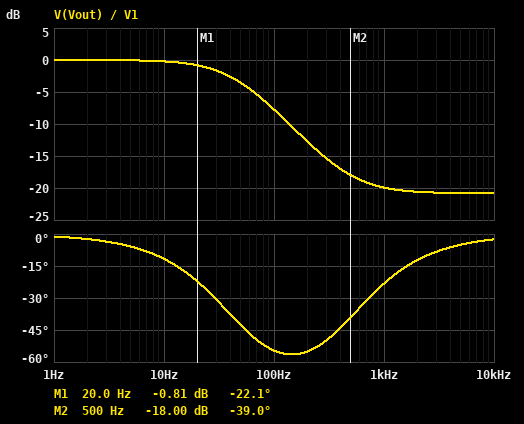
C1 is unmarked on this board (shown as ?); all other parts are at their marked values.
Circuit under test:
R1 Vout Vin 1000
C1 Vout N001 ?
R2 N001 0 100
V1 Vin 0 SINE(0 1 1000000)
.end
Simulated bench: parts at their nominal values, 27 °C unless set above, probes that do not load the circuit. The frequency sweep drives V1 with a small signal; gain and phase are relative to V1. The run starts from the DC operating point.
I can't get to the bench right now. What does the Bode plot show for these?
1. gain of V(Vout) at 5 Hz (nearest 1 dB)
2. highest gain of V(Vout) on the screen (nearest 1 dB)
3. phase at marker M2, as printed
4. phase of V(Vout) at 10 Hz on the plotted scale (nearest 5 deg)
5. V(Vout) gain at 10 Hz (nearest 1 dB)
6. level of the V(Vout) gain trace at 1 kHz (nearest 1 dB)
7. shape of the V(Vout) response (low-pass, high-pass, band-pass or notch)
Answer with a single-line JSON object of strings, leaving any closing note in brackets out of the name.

{"gain of V(Vout) at 5 Hz": "0 dB", "highest gain of V(Vout) on the screen": "0 dB", "phase at marker M2, as printed": "-39.0 deg", "phase of V(Vout) at 10 Hz on the plotted scale": "-10 deg", "V(Vout) gain at 10 Hz": "0 dB", "level of the V(Vout) gain trace at 1 kHz": "-20 dB", "shape of the V(Vout) response": "low-pass"}
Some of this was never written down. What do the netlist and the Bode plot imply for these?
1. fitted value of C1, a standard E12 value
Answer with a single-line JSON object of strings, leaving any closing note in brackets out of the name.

{"fitted value of C1, a standard E12 value": "3.3 µF"}
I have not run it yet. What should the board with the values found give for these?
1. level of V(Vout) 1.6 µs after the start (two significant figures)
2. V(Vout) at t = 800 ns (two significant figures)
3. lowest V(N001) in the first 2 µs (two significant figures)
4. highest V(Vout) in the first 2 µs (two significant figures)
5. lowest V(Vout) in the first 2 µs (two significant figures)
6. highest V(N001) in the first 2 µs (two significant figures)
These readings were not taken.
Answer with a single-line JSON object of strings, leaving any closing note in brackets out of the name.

{"level of V(Vout) 1.6 µs after the start": "-53 mV", "V(Vout) at t = 800 ns": "-86 mV", "lowest V(N001) in the first 2 µs": "-91 mV", "highest V(Vout) in the first 2 µs": "91 mV", "lowest V(Vout) in the first 2 µs": "-91 mV", "highest V(N001) in the first 2 µs": "91 mV"}
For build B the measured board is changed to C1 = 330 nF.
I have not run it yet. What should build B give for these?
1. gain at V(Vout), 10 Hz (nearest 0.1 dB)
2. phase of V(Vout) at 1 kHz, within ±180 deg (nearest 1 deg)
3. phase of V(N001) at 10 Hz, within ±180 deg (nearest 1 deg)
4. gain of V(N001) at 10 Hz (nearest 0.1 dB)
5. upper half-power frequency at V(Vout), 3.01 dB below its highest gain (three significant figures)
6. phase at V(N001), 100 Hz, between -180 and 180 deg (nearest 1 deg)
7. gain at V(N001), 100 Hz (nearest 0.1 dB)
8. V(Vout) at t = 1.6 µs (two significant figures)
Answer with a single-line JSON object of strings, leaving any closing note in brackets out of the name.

{"gain at V(Vout), 10 Hz": "0 dB", "phase of V(Vout) at 1 kHz, within ±180 deg": "-55 deg", "phase of V(N001) at 10 Hz, within ±180 deg": "89 deg", "gain of V(N001) at 10 Hz": "-53.7 dB", "upper half-power frequency at V(Vout), 3.01 dB below its highest gain": "442 Hz", "phase at V(N001), 100 Hz, between -180 and 180 deg": "77 deg", "gain at V(N001), 100 Hz": "-33.9 dB", "V(Vout) at t = 1.6 µs": "-53 mV"}
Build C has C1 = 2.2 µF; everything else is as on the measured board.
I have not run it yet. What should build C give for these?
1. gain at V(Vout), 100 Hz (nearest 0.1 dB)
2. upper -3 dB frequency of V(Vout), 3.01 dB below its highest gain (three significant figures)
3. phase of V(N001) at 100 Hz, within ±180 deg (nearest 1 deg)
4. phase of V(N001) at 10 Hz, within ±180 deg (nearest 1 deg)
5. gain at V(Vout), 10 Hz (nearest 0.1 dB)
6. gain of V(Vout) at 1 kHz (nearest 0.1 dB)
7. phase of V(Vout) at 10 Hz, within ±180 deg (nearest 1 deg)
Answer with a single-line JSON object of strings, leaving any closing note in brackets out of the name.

{"gain at V(Vout), 100 Hz": "-5.1 dB", "upper -3 dB frequency of V(Vout), 3.01 dB below its highest gain": "66.3 Hz", "phase of V(N001) at 100 Hz, within ±180 deg": "33 deg", "phase of V(N001) at 10 Hz, within ±180 deg": "81 deg", "gain at V(Vout), 10 Hz": "-0.1 dB", "gain of V(Vout) at 1 kHz": "-19.0 dB", "phase of V(Vout) at 10 Hz, within ±180 deg": "-8 deg"}
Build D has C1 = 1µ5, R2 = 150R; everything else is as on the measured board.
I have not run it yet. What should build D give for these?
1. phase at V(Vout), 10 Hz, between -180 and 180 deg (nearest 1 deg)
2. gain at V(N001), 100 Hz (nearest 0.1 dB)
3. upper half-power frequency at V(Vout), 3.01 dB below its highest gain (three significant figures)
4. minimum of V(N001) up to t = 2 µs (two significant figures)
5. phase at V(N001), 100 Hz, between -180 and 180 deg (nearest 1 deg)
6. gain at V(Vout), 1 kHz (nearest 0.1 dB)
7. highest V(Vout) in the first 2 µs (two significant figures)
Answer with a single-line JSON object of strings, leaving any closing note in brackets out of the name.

{"phase at V(Vout), 10 Hz, between -180 and 180 deg": "-5 deg", "gain at V(N001), 100 Hz": "-20.4 dB", "upper half-power frequency at V(Vout), 3.01 dB below its highest gain": "93.9 Hz", "minimum of V(N001) up to t = 2 µs": "-130 mV", "phase at V(N001), 100 Hz, between -180 and 180 deg": "43 deg", "gain at V(Vout), 1 kHz": "-16.0 dB", "highest V(Vout) in the first 2 µs": "130 mV"}
